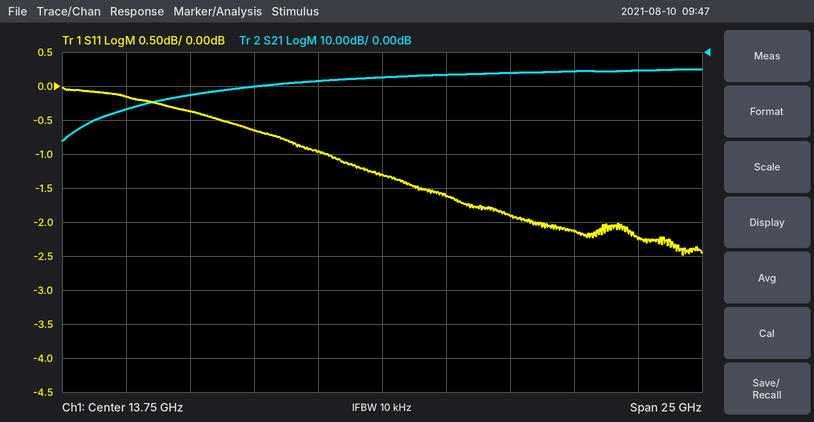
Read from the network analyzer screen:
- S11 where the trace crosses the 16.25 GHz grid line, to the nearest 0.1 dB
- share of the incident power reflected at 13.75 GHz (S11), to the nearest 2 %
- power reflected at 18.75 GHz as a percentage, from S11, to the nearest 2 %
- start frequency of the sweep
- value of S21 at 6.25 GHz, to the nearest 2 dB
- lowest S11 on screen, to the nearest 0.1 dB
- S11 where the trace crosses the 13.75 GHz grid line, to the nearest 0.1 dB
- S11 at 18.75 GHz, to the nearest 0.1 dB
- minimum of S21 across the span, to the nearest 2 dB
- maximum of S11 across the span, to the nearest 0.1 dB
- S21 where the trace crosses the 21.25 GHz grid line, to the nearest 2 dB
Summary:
-1.6 dB
74 %
64 %
1.25 GHz
-12 dB
-2.5 dB
-1.3 dB
-1.9 dB
-26 dB
0.0 dB
-6 dB
